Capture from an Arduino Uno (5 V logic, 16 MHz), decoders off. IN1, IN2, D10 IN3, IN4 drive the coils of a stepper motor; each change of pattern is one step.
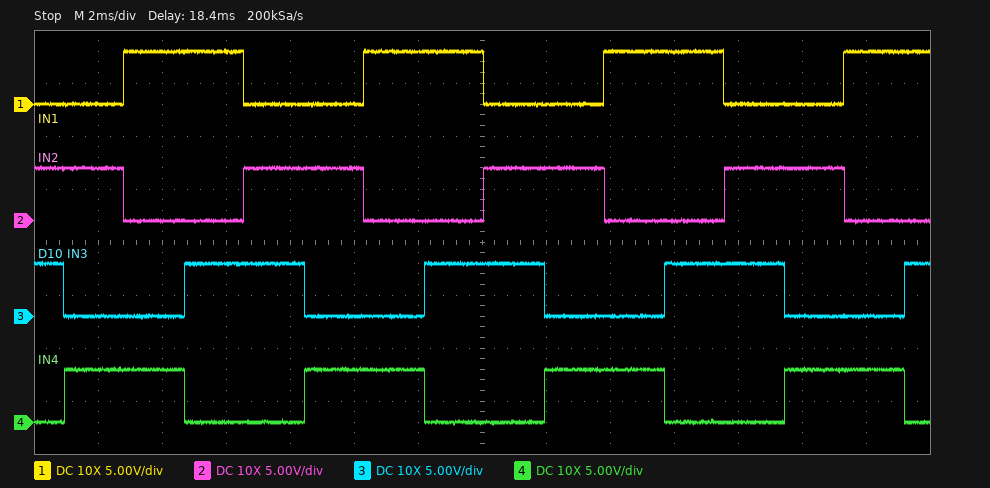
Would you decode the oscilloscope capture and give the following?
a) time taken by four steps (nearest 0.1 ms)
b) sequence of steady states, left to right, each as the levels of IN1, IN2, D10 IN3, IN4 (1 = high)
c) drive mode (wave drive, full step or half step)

7.5 ms
0110 0101 1001 1010 0110 0101 1001 1010 0110 0101 1001 1010 0110 0101 1001 1010
full step
